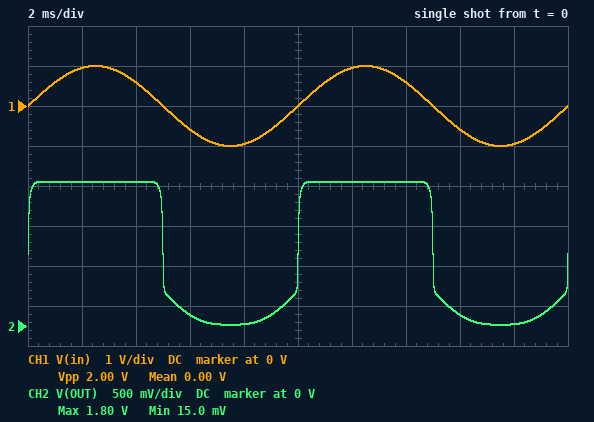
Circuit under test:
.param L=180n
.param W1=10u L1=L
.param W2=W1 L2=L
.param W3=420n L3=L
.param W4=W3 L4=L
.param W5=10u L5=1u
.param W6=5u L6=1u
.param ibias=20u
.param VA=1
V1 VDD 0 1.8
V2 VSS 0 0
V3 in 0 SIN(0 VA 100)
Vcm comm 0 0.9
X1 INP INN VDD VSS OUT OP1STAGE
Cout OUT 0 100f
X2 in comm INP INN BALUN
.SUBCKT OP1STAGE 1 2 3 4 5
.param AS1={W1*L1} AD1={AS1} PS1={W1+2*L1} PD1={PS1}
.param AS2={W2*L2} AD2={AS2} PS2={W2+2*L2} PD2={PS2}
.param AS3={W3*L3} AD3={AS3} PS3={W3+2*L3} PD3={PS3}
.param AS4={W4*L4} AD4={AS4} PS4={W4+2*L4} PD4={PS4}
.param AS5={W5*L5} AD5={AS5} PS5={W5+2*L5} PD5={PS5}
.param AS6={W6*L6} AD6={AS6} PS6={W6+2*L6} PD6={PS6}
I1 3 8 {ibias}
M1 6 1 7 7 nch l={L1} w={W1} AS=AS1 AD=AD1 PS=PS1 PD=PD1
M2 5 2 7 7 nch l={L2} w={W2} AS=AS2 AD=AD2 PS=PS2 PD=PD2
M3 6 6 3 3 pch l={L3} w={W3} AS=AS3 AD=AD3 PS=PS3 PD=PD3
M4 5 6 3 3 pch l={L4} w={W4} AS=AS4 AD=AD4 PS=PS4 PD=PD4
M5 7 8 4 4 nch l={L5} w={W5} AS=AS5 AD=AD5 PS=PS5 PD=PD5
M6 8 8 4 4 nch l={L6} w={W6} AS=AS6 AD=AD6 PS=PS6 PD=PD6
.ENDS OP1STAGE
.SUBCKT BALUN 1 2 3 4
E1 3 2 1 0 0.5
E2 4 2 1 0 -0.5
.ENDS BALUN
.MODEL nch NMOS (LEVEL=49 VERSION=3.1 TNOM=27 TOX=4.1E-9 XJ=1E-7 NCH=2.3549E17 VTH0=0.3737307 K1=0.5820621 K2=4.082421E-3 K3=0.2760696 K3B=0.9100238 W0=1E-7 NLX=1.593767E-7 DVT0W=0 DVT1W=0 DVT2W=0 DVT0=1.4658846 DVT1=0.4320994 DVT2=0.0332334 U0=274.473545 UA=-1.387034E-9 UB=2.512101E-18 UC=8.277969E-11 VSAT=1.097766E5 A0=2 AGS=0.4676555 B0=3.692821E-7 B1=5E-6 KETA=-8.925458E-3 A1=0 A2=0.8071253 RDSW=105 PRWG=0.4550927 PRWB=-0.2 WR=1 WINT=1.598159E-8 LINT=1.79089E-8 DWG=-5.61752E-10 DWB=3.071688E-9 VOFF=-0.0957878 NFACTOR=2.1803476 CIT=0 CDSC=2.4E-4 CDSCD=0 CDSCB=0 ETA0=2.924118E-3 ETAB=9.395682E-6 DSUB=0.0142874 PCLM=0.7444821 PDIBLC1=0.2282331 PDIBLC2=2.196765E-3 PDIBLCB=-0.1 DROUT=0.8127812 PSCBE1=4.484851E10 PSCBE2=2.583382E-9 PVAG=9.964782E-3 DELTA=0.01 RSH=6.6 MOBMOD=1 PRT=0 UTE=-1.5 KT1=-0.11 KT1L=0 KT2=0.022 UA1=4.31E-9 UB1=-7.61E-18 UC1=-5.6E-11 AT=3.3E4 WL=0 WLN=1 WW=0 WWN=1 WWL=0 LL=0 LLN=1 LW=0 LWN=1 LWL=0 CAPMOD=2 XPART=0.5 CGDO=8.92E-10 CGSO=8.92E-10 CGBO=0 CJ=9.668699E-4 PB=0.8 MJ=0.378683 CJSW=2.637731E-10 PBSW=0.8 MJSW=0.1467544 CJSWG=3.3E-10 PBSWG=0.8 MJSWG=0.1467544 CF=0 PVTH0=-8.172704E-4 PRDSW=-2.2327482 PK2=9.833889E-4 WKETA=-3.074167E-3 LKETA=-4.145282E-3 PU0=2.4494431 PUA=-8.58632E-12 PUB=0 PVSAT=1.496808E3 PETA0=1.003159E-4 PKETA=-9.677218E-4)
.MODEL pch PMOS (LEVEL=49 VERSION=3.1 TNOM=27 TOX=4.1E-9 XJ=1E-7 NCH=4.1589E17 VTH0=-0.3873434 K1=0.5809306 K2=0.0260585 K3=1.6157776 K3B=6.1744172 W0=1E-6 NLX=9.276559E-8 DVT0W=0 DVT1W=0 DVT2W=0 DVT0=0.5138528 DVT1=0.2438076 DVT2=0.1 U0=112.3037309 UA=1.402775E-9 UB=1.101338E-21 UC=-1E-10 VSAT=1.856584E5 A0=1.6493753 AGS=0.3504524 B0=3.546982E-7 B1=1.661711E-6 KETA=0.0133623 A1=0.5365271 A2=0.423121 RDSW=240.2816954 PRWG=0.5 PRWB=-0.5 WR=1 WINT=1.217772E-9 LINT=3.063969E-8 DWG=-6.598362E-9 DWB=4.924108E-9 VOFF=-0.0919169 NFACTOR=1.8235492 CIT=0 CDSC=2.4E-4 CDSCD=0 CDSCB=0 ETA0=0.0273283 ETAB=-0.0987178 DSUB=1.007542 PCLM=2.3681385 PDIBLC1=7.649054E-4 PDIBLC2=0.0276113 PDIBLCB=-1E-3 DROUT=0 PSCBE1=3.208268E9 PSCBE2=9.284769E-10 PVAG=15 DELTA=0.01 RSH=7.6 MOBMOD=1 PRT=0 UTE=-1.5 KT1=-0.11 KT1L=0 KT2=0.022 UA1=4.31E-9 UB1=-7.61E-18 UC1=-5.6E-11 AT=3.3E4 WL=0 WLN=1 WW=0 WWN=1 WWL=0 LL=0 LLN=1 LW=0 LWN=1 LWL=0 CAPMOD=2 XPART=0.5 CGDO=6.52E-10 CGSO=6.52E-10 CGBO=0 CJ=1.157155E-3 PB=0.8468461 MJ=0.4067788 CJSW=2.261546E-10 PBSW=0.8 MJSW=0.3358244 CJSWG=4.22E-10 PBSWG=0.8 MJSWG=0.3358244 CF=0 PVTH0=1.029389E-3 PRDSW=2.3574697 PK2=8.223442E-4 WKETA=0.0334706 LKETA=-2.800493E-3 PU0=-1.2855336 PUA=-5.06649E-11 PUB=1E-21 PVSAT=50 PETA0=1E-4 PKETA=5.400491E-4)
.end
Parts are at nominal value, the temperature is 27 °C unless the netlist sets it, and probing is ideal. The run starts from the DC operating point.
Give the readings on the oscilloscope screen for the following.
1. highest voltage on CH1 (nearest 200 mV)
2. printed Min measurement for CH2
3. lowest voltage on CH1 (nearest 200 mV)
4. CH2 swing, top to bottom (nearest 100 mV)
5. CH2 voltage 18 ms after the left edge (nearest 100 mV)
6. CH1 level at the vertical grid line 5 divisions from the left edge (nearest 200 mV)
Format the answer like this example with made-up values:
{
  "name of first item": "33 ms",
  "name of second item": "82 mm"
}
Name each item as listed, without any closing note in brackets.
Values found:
{
  "highest voltage on CH1": "1.0 V",
  "printed Min measurement for CH2": "15.0 mV",
  "lowest voltage on CH1": "-1.0 V",
  "CH2 swing, top to bottom": "1.8 V",
  "CH2 voltage 18 ms after the left edge": "0 V",
  "CH1 level at the vertical grid line 5 divisions from the left edge": "0 V"
}
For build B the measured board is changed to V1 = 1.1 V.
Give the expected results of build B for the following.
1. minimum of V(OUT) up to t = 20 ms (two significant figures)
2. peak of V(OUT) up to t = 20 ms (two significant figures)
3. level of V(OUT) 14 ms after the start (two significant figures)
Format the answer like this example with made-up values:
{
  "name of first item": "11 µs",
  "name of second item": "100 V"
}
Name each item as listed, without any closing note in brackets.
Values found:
{
  "minimum of V(OUT) up to t = 20 ms": "10 mV",
  "peak of V(OUT) up to t = 20 ms": "1.1 V",
  "level of V(OUT) 14 ms after the start": "940 mV"
}
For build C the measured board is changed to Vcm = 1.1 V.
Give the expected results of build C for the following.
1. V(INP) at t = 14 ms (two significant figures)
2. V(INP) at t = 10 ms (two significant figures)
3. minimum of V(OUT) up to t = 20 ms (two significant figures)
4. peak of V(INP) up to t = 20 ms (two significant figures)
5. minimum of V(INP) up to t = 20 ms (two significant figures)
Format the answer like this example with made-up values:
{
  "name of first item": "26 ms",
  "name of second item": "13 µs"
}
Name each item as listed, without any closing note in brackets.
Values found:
{
  "V(INP) at t = 14 ms": "1.4 V",
  "V(INP) at t = 10 ms": "1.1 V",
  "minimum of V(OUT) up to t = 20 ms": "130 mV",
  "peak of V(INP) up to t = 20 ms": "1.6 V",
  "minimum of V(INP) up to t = 20 ms": "600 mV"
}
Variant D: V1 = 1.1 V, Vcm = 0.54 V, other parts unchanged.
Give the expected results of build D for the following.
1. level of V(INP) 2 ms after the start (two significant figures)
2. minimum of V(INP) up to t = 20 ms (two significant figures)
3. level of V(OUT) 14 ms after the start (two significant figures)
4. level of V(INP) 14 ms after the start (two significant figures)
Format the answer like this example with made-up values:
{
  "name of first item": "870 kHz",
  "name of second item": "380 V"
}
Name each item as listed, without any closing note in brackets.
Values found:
{
  "level of V(INP) 2 ms after the start": "1.0 V",
  "minimum of V(INP) up to t = 20 ms": "40 mV",
  "level of V(OUT) 14 ms after the start": "1.1 V",
  "level of V(INP) 14 ms after the start": "830 mV"
}
